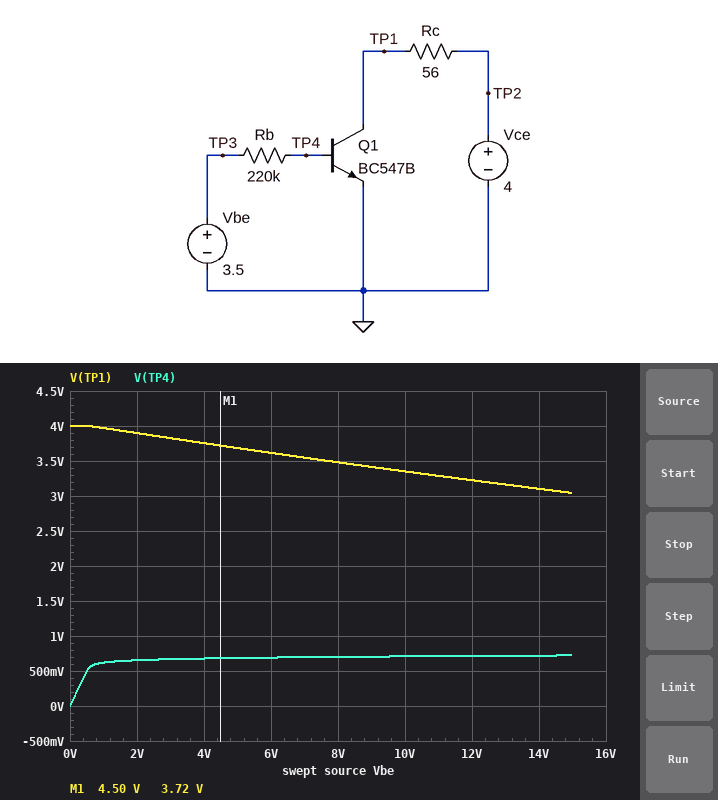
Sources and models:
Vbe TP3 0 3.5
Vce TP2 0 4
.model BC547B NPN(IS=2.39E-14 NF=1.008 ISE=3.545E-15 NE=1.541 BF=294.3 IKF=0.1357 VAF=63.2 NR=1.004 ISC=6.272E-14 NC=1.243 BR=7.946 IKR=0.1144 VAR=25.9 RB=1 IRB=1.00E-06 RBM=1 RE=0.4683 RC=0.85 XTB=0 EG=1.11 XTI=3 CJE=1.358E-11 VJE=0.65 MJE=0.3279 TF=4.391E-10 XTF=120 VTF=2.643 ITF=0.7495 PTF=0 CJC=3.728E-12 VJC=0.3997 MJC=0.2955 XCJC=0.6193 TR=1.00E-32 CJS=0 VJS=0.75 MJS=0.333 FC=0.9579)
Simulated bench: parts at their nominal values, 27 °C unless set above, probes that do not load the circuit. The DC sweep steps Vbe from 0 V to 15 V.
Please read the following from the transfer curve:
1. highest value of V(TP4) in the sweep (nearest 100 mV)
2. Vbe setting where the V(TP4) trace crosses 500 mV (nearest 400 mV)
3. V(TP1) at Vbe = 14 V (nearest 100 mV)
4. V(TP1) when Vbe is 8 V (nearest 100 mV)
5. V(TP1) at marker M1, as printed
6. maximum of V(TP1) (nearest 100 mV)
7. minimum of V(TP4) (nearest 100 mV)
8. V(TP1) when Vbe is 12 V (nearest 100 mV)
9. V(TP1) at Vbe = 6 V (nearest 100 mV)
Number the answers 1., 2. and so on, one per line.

1. 700 mV
2. 400 mV
3. 3.1 V
4. 3.5 V
5. 3.72 V
6. 4.0 V
7. 0 V
8. 3.2 V
9. 3.6 V
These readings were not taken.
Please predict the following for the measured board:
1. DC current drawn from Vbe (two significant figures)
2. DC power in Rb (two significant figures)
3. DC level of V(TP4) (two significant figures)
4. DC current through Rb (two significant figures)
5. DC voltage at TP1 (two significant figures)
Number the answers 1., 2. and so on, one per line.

1. 13 µA
2. 36 µW
3. 670 mV
4. 13 µA
5. 3.8 V
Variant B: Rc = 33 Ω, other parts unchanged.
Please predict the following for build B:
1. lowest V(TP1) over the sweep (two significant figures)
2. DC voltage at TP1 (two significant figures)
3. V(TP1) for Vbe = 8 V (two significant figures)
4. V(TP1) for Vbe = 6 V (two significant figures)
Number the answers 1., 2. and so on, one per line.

1. 3.4 V
2. 3.9 V
3. 3.7 V
4. 3.8 V
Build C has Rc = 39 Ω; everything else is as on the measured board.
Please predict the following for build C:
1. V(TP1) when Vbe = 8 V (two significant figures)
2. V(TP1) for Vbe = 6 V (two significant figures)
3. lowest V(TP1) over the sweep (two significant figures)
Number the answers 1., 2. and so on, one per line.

1. 3.6 V
2. 3.7 V
3. 3.3 V
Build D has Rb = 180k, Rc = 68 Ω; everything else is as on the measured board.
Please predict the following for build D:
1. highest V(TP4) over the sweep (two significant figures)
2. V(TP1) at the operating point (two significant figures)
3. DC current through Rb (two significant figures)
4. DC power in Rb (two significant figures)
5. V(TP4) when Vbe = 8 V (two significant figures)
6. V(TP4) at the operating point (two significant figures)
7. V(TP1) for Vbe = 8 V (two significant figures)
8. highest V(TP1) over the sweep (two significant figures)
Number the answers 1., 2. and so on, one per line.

1. 730 mV
2. 3.7 V
3. 16 µA
4. 44 µW
5. 710 mV
6. 680 mV
7. 3.2 V
8. 4.0 V
